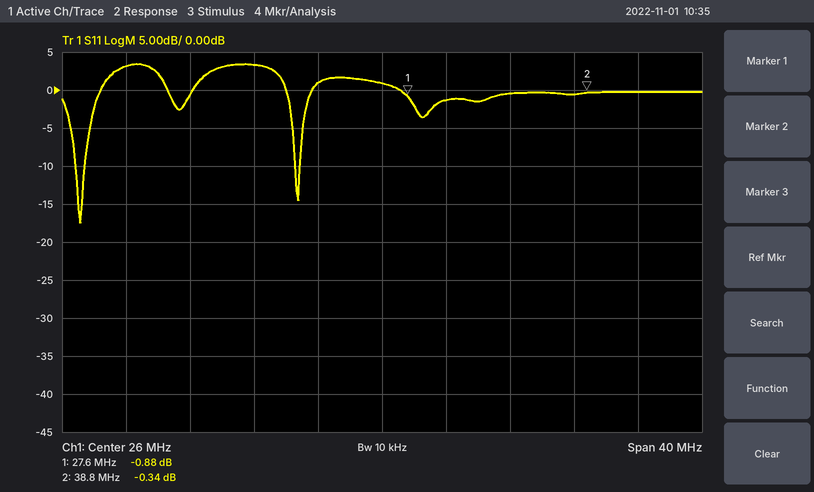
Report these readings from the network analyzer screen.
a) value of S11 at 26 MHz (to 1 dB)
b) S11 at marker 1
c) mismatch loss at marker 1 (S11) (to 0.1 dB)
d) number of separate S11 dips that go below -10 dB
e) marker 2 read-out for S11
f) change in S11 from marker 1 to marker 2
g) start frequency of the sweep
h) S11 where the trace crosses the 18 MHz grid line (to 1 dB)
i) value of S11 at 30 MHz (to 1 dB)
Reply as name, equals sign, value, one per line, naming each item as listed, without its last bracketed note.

value of S11 at 26 MHz = 1 dB
S11 at marker 1 = -0.88 dB
mismatch loss at marker 1 (S11) = 7.4 dB
number of separate S11 dips that go below -10 dB = 2
marker 2 read-out for S11 = -0.34 dB
change in S11 from marker 1 to marker 2 = 0.54 dB
start frequency of the sweep = 6 MHz
S11 where the trace crosses the 18 MHz grid line = 3 dB
value of S11 at 30 MHz = -1 dB
